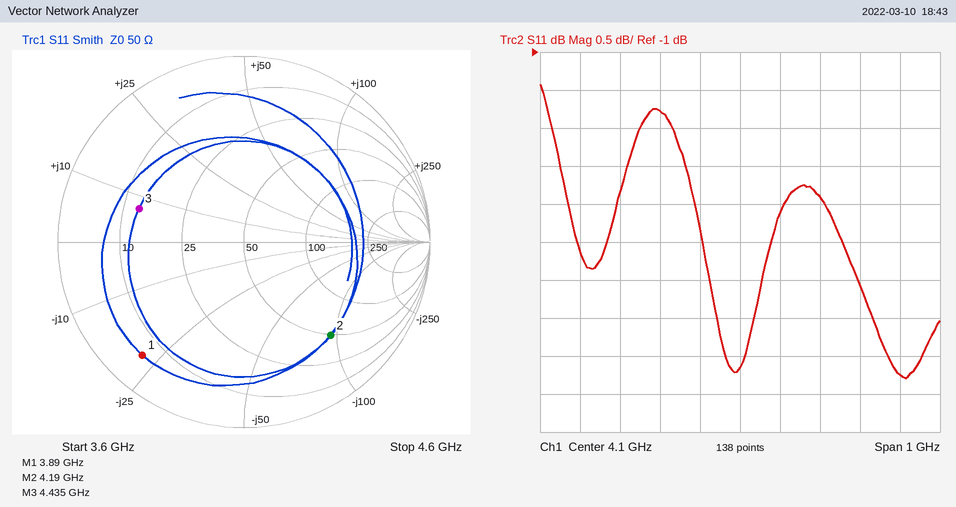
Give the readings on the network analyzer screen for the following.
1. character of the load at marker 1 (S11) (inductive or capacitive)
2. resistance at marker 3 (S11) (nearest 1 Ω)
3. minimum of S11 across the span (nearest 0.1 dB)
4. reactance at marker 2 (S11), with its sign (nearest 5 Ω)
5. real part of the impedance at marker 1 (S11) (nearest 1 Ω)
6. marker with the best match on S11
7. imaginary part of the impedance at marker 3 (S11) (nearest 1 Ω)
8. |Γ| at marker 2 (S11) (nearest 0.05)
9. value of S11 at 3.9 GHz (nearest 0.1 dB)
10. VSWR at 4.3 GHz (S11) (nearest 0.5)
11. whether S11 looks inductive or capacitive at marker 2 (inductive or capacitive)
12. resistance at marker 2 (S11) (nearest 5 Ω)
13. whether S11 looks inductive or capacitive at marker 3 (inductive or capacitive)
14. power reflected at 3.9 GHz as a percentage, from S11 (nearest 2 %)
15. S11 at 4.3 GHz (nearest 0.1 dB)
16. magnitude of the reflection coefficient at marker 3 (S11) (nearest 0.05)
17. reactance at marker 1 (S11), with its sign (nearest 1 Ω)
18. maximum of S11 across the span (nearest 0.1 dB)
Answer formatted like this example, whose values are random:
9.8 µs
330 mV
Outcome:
capacitive
13 Ω
-5.3 dB
-95 Ω
6 Ω
marker 3
+7 Ω
0.70
-1.8 dB
6.0
capacitive
50 Ω
inductive
66 %
-2.9 dB
0.60
-22 Ω
-1.4 dB
